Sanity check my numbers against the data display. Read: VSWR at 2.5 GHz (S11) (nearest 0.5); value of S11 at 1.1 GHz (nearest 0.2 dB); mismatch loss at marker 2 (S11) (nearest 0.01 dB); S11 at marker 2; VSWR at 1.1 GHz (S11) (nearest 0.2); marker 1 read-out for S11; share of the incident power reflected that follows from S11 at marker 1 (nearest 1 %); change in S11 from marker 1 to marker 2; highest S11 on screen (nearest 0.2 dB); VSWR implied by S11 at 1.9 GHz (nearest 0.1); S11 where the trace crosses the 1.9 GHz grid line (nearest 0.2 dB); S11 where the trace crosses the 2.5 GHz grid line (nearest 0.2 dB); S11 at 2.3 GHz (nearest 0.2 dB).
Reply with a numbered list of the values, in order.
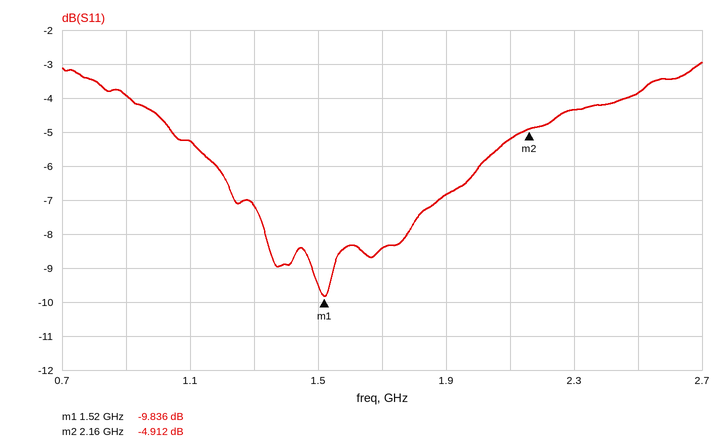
1. 4.5
2. -5.2 dB
3. 1.69 dB
4. -4.912 dB
5. 3.4
6. -9.836 dB
7. 10 %
8. 4.924 dB
9. -3.0 dB
10. 2.7
11. -6.8 dB
12. -3.8 dB
13. -4.4 dB
